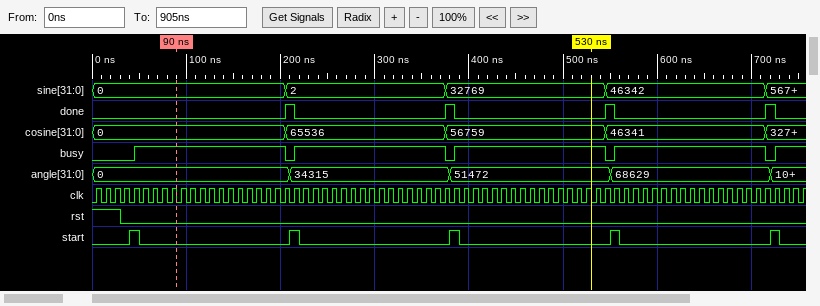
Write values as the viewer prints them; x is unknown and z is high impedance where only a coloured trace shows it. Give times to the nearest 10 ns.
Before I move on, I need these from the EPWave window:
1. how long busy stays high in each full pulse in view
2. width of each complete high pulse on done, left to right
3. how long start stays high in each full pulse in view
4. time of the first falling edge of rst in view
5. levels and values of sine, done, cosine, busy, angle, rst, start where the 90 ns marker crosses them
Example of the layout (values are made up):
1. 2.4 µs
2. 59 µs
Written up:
1. 160 ns, 160 ns, 160 ns, 160 ns
2. 10 ns, 10 ns, 10 ns, 10 ns
3. 10 ns, 10 ns, 10 ns, 10 ns, 10 ns
4. 30 ns
5. sine=0, done=0, cosine=0, busy=1, angle=0, rst=0, start=0
